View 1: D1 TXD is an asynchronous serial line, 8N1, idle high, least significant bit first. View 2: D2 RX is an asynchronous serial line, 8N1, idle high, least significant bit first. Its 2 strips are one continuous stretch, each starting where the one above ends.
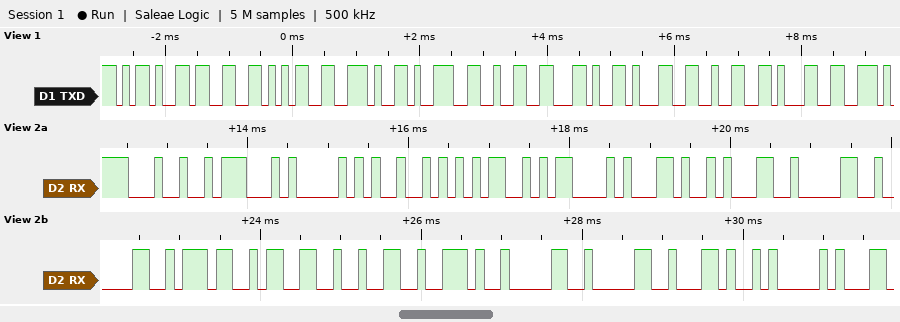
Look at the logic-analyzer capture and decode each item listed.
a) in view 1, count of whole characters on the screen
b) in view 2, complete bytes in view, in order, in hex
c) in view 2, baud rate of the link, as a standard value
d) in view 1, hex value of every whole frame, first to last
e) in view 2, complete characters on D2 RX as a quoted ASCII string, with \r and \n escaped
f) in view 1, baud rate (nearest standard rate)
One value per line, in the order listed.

10
24 47 50 52 4D 43 2C 31 30 30 37 33 32 2E 30 30 2C 41
9600 baud
2D 33 35 2E 39 32 2C 31 32 31
"$GPRMC,100732.00,A"
9600 baud
